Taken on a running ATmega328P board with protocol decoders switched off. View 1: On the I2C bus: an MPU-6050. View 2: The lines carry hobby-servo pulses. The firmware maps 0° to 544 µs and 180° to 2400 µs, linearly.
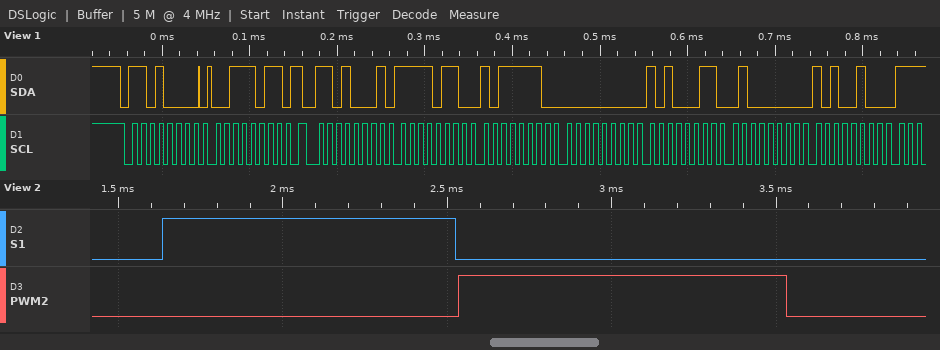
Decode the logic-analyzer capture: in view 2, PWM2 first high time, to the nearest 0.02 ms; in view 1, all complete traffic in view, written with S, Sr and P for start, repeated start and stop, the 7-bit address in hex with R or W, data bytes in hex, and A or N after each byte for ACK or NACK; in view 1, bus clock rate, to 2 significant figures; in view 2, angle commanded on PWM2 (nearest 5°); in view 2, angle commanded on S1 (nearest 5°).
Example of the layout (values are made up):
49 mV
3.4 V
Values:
1.00 ms
S 68W A 3B A Sr 68R A F6 A BE A 00 A A3 A 40 A A4 A
100 kHz
45°
35°
